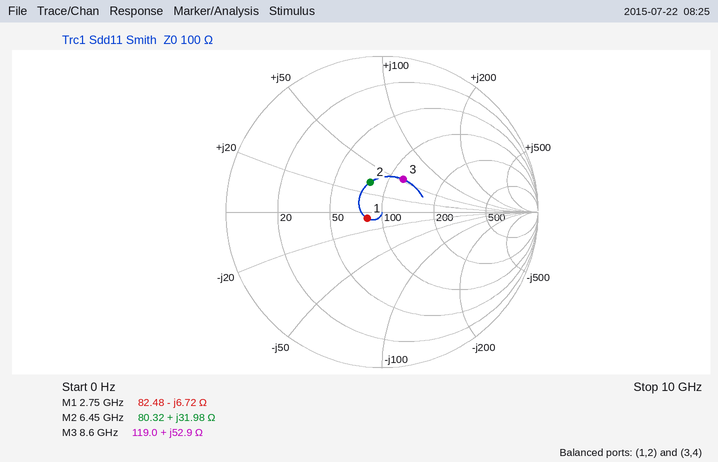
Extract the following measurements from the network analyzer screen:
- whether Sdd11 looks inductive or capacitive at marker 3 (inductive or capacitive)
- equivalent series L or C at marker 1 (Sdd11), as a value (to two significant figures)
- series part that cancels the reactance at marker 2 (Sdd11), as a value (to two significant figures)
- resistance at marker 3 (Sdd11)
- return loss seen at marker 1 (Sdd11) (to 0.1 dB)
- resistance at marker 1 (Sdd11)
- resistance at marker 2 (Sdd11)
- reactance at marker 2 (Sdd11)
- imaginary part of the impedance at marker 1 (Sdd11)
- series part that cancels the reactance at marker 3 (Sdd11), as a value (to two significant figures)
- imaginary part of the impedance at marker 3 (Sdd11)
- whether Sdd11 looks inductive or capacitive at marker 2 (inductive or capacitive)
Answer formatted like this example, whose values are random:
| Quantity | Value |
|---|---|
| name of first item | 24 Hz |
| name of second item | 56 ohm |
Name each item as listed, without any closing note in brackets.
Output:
| Quantity | Value |
|---|---|
| whether Sdd11 looks inductive or capacitive at marker 3 | inductive |
| equivalent series L or C at marker 1 (Sdd11), as a value | 8.6 pF |
| series part that cancels the reactance at marker 2 (Sdd11), as a value | 770 fF |
| resistance at marker 3 | 119.0 Ω |
| return loss seen at marker 1 (Sdd11) | 19.8 dB |
| resistance at marker 1 | 82.48 Ω |
| resistance at marker 2 | 80.32 Ω |
| reactance at marker 2 | +31.98 Ω |
| imaginary part of the impedance at marker 1 | -6.72 Ω |
| series part that cancels the reactance at marker 3 (Sdd11), as a value | 350 fF |
| imaginary part of the impedance at marker 3 | +52.9 Ω |
| whether Sdd11 looks inductive or capacitive at marker 2 | inductive |
